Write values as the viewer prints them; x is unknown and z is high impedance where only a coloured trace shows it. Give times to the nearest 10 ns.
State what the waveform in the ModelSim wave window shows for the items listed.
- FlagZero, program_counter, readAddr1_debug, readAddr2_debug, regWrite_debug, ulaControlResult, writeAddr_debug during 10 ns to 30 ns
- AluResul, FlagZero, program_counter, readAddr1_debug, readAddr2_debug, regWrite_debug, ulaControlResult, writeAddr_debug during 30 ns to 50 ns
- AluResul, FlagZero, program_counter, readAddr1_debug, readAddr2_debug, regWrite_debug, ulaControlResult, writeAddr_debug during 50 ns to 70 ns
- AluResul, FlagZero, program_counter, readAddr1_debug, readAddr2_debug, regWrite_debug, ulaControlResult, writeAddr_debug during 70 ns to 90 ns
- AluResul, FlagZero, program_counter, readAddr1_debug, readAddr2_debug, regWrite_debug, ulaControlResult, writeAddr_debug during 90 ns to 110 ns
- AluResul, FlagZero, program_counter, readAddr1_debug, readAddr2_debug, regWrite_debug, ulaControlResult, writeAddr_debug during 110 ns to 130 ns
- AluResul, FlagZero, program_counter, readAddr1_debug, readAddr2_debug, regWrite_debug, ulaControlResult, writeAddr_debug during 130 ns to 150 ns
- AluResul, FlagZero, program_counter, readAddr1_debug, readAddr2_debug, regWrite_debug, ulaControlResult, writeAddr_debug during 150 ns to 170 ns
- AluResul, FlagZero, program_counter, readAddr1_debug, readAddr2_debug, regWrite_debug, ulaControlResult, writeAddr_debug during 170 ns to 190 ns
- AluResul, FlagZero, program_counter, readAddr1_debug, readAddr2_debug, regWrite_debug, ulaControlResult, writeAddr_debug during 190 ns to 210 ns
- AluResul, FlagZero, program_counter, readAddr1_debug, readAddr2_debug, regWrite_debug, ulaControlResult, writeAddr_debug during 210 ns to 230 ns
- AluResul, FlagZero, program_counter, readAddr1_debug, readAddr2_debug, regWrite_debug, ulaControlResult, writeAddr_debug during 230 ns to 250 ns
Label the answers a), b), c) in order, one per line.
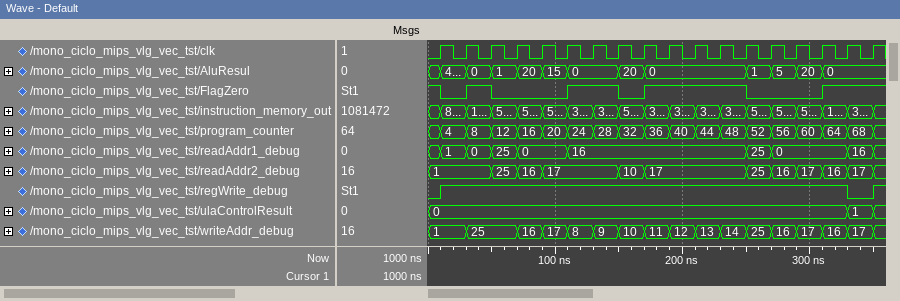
a) FlagZero=0, program_counter=4, readAddr1_debug=1, readAddr2_debug=1, regWrite_debug=1, ulaControlResult=0, writeAddr_debug=1
b) AluResul=0, FlagZero=1, program_counter=8, readAddr1_debug=0, readAddr2_debug=1, regWrite_debug=1, ulaControlResult=0, writeAddr_debug=25
c) AluResul=1, FlagZero=0, program_counter=12, readAddr1_debug=25, readAddr2_debug=25, regWrite_debug=1, ulaControlResult=0, writeAddr_debug=25
d) AluResul=20, FlagZero=0, program_counter=16, readAddr1_debug=0, readAddr2_debug=16, regWrite_debug=1, ulaControlResult=0, writeAddr_debug=16
e) AluResul=15, FlagZero=0, program_counter=20, readAddr1_debug=0, readAddr2_debug=17, regWrite_debug=1, ulaControlResult=0, writeAddr_debug=17
f) AluResul=0, FlagZero=1, program_counter=24, readAddr1_debug=16, readAddr2_debug=17, regWrite_debug=1, ulaControlResult=0, writeAddr_debug=8
g) AluResul=0, FlagZero=1, program_counter=28, readAddr1_debug=16, readAddr2_debug=17, regWrite_debug=1, ulaControlResult=0, writeAddr_debug=9
h) AluResul=20, FlagZero=0, program_counter=32, readAddr1_debug=16, readAddr2_debug=10, regWrite_debug=1, ulaControlResult=0, writeAddr_debug=10
i) AluResul=0, FlagZero=1, program_counter=36, readAddr1_debug=16, readAddr2_debug=17, regWrite_debug=1, ulaControlResult=0, writeAddr_debug=11
j) AluResul=0, FlagZero=1, program_counter=40, readAddr1_debug=16, readAddr2_debug=17, regWrite_debug=1, ulaControlResult=0, writeAddr_debug=12
k) AluResul=0, FlagZero=1, program_counter=44, readAddr1_debug=16, readAddr2_debug=17, regWrite_debug=1, ulaControlResult=0, writeAddr_debug=13
l) AluResul=0, FlagZero=1, program_counter=48, readAddr1_debug=16, readAddr2_debug=17, regWrite_debug=1, ulaControlResult=0, writeAddr_debug=14
